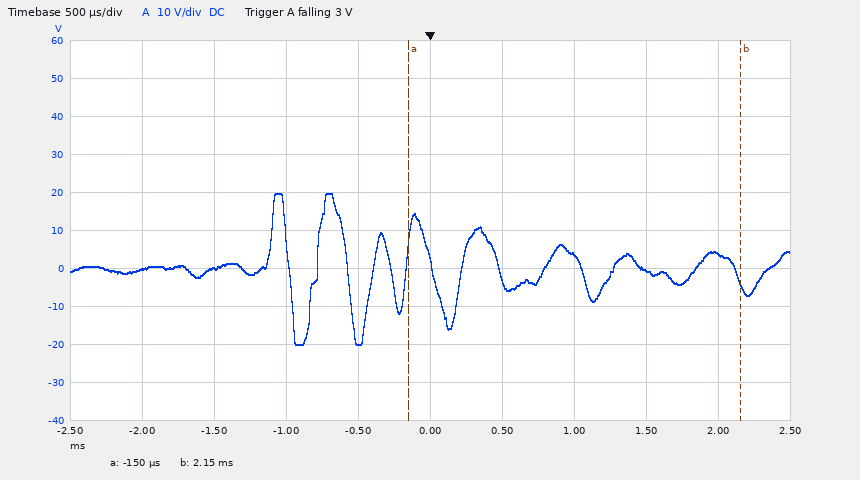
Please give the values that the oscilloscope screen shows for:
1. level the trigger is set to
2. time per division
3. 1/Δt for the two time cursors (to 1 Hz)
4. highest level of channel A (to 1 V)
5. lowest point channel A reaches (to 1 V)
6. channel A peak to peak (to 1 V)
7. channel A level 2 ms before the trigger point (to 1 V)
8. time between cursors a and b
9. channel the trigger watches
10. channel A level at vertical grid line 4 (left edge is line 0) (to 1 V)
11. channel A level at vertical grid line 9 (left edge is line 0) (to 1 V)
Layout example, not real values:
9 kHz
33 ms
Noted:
3 V
500 µs
435 Hz
20 V
-20 V
40 V
0 V
2.30 ms
channel A
-19 V
4 V
